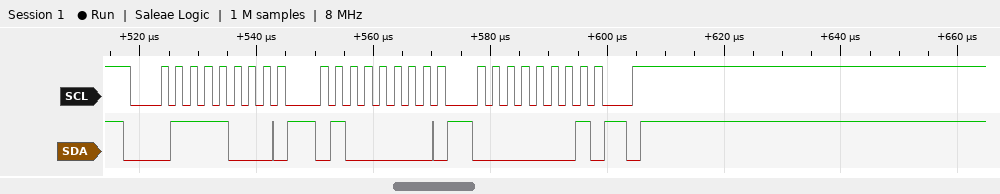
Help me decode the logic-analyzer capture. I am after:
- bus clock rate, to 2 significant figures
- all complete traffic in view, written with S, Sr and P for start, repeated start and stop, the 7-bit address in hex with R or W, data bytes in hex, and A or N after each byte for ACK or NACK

400 kHz
S 3CW A 40 A 01 A P
